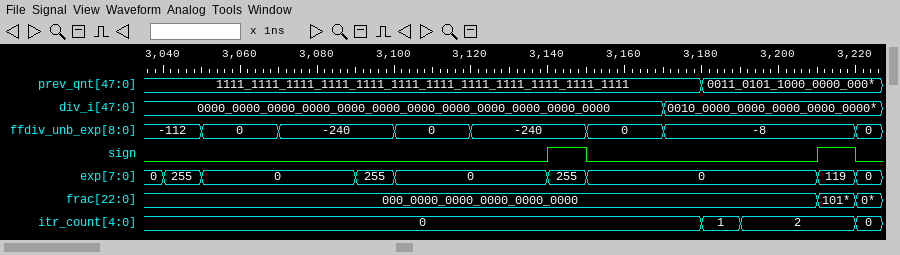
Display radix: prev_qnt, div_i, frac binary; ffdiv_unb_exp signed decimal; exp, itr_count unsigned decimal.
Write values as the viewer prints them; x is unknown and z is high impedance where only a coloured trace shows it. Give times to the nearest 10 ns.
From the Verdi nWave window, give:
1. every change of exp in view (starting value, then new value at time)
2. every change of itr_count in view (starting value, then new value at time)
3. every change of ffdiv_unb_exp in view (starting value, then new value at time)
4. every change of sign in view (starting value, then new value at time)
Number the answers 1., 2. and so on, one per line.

1. 0, 255 at 3040 ns, 0 at 3050 ns, 255 at 3090 ns, 0 at 3100 ns, 255 at 3140 ns, 0 at 3150 ns, 119 at 3210 ns, 0 at 3220 ns
2. 0, 1 at 3180 ns, 2 at 3190 ns, 0 at 3220 ns
3. -112, 0 at 3050 ns, -240 at 3070 ns, 0 at 3100 ns, -240 at 3120 ns, 0 at 3150 ns, -8 at 3170 ns, 0 at 3220 ns
4. 0, 1 at 3140 ns, 0 at 3150 ns, 1 at 3210 ns, 0 at 3220 ns
